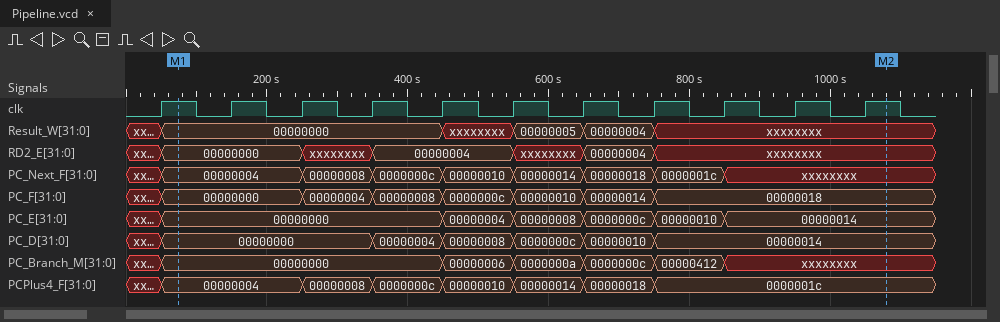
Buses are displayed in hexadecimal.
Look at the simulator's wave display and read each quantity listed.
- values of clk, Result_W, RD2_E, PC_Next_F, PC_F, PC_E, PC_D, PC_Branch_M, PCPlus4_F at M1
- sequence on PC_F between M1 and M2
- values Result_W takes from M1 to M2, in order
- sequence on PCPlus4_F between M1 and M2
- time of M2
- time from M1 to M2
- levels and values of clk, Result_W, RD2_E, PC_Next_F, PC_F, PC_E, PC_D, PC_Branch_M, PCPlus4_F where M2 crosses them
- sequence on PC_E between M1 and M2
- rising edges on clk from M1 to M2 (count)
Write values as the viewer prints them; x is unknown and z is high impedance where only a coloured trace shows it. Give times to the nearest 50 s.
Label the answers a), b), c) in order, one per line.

a) clk=1, Result_W=00000000, RD2_E=00000000, PC_Next_F=00000004, PC_F=00000000, PC_E=00000000, PC_D=00000000, PC_Branch_M=00000000, PCPlus4_F=00000004
b) 00000000, 00000004, 00000008, 0000000c, 00000010, 00000014, 00000018
c) 00000000, xxxxxxxx, 00000005, 00000004, xxxxxxxx
d) 00000004, 00000008, 0000000c, 00000010, 00000014, 00000018, 0000001c
e) 1100 s
f) 1000 s
g) clk=1, Result_W=xxxxxxxx, RD2_E=xxxxxxxx, PC_Next_F=xxxxxxxx, PC_F=00000018, PC_E=00000014, PC_D=00000014, PC_Branch_M=xxxxxxxx, PCPlus4_F=0000001c
h) 00000000, 00000004, 00000008, 0000000c, 00000010, 00000014
i) 10
